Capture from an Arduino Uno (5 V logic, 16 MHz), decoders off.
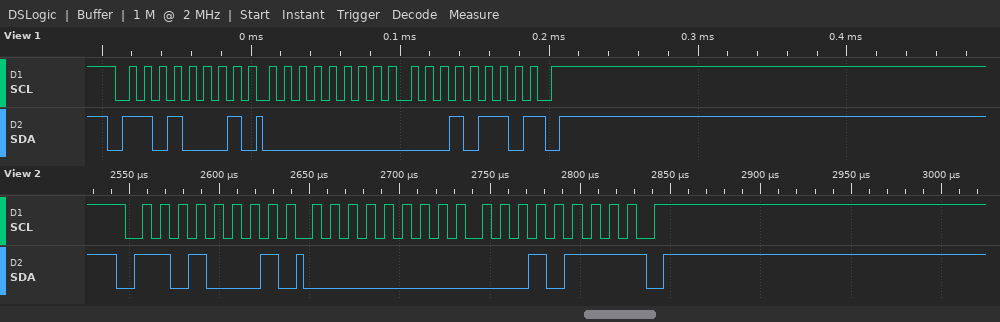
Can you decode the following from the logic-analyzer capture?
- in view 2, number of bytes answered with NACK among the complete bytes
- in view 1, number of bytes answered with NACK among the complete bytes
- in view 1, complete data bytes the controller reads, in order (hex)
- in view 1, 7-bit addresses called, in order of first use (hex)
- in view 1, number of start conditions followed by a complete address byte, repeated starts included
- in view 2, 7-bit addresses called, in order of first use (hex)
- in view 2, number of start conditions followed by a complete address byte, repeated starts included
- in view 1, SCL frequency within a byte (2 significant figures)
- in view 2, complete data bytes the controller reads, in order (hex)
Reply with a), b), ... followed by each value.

a) 1
b) 1
c) 00 16
d) 0x68
e) 1
f) 0x68
g) 1
h) 100 kHz
i) 00 17
